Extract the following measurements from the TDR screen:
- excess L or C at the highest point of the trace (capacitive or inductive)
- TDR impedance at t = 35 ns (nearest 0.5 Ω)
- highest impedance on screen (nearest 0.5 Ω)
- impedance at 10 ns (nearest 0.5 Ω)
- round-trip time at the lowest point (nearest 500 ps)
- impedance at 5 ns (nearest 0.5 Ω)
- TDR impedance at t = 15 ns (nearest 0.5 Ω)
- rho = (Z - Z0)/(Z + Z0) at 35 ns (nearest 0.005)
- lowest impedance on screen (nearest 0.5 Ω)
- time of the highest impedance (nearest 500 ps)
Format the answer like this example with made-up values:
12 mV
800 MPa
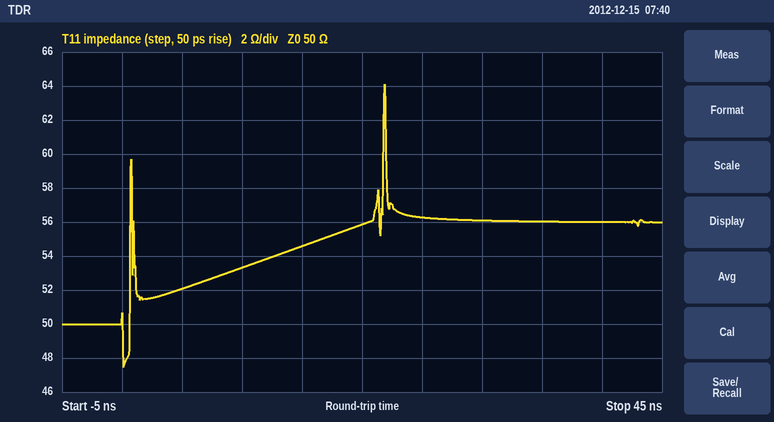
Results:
inductive
56.0 Ω
64.0 Ω
53.5 Ω
0.0 ns
52.0 Ω
54.5 Ω
+0.055
47.5 Ω
22.0 ns
